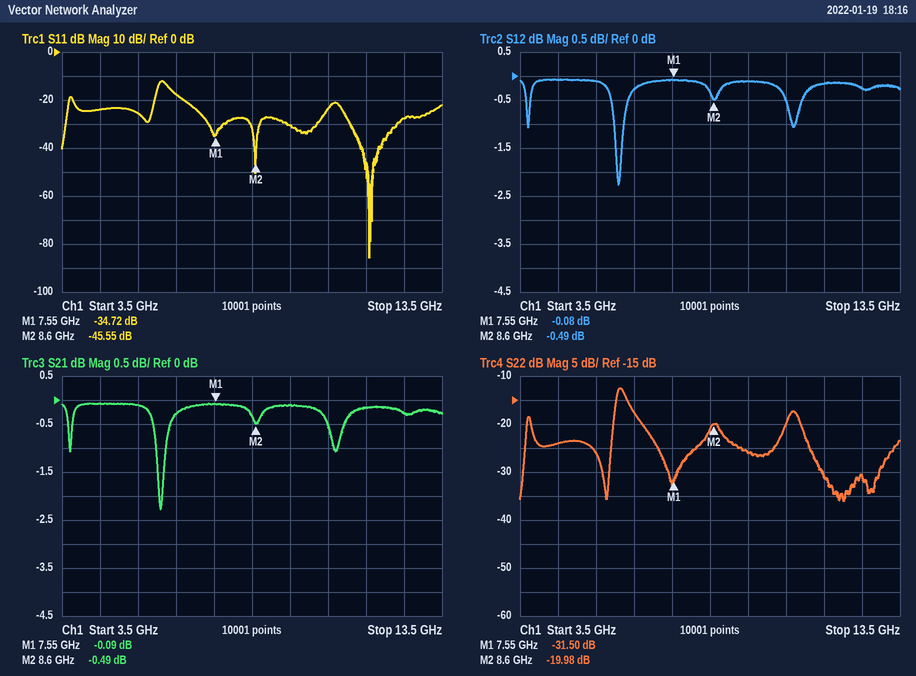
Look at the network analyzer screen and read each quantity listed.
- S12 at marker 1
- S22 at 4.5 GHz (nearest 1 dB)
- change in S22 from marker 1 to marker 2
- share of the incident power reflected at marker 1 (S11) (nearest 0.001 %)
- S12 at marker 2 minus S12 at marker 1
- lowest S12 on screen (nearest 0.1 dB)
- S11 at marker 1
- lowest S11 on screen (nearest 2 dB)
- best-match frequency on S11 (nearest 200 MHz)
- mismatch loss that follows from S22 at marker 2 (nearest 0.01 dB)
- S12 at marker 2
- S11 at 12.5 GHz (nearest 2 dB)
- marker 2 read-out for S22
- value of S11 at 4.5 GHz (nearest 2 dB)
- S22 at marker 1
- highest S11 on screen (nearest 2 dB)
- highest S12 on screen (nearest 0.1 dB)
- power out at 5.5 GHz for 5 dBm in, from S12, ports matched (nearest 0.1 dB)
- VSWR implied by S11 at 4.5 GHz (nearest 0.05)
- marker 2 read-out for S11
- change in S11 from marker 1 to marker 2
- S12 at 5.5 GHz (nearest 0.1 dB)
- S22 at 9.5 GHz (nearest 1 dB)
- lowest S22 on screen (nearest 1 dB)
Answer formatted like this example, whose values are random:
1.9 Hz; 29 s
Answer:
-0.08 dB; -24 dB; 11.52 dB; 0.034 %; -0.41 dB; -2.3 dB; -34.72 dB; -86 dB; 11.6 GHz; 0.04 dB; -0.49 dB; -28 dB; -19.98 dB; -24 dB; -31.50 dB; -12 dB; -0.1 dB; 4.9 dBm; 1.15; -45.55 dB; -10.83 dB; -0.1 dB; -26 dB; -36 dB
